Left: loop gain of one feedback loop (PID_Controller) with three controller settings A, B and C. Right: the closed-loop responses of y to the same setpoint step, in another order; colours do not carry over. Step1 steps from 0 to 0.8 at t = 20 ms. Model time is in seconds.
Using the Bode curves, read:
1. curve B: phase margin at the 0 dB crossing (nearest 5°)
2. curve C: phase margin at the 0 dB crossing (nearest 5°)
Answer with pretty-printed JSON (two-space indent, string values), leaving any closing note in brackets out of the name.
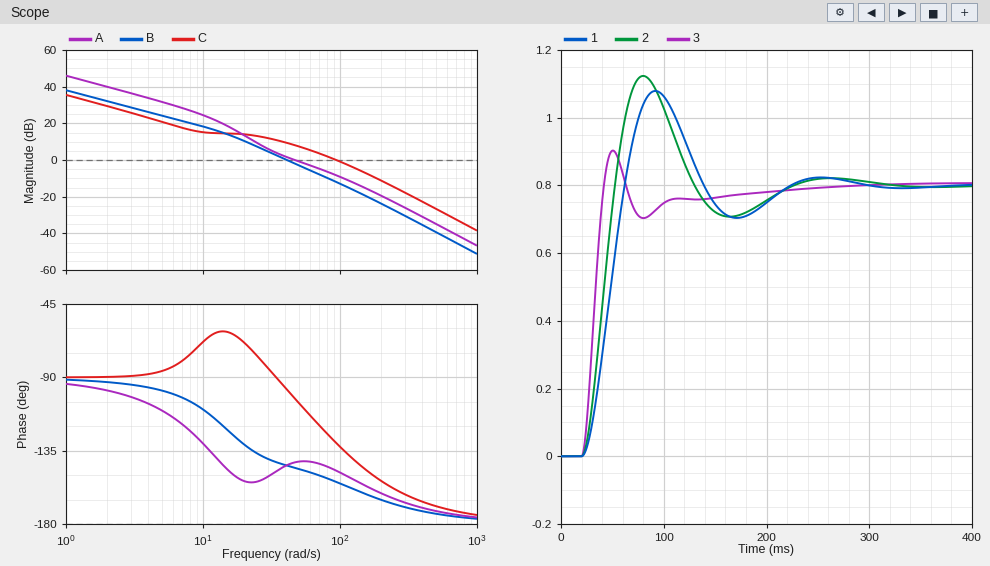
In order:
{
  "curve B: phase margin at the 0 dB crossing": "35°",
  "curve C: phase margin at the 0 dB crossing": "50°"
}
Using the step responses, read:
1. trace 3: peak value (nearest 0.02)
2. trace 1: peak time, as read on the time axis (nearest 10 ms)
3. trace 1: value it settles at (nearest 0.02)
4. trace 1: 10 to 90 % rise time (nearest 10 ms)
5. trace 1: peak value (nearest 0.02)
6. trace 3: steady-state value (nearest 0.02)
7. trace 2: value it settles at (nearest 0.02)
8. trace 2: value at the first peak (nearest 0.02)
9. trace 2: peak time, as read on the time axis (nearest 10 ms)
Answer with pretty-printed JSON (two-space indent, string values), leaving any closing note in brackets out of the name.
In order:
{
  "trace 3: peak value": "0.90",
  "trace 1: peak time, as read on the time axis": "90 ms",
  "trace 1: value it settles at": "0.80",
  "trace 1: 10 to 90 % rise time": "30 ms",
  "trace 1: peak value": "1.08",
  "trace 3: steady-state value": "0.80",
  "trace 2: value it settles at": "0.80",
  "trace 2: value at the first peak": "1.12",
  "trace 2: peak time, as read on the time axis": "80 ms"
}
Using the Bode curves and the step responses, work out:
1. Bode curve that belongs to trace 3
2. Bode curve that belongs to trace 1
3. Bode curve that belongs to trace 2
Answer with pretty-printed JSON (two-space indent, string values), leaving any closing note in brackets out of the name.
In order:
{
  "Bode curve that belongs to trace 3": "C",
  "Bode curve that belongs to trace 1": "B",
  "Bode curve that belongs to trace 2": "A"
}
